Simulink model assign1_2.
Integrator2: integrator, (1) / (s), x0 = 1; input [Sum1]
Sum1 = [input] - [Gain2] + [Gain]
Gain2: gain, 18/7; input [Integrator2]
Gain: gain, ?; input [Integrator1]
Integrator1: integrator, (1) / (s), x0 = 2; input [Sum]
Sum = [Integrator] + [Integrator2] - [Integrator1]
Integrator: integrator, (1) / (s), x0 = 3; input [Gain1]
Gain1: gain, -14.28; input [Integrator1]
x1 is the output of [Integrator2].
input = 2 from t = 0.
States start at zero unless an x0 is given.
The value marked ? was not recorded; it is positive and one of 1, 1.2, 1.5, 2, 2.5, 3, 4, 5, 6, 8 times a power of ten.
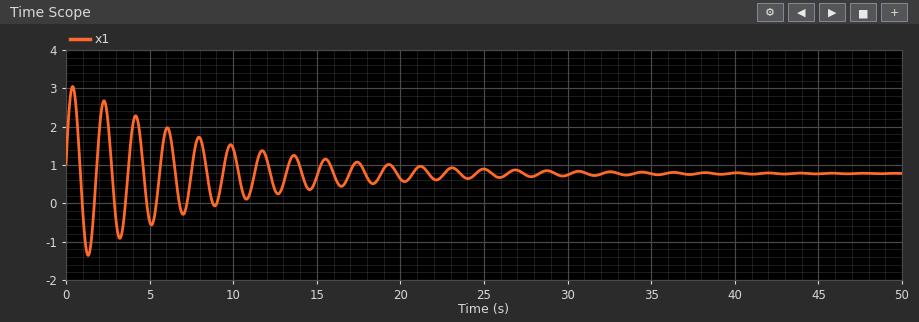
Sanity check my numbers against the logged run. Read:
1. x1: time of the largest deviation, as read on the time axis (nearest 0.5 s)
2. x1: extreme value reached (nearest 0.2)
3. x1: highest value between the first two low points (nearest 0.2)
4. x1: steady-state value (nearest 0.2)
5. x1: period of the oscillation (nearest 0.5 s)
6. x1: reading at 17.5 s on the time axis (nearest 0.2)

1.5 s
-1.4
2.6
0.8
2.0 s
1.0
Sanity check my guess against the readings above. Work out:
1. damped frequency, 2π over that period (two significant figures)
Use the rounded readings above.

3.1 rad/s
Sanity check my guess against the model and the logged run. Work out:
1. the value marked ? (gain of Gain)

5
